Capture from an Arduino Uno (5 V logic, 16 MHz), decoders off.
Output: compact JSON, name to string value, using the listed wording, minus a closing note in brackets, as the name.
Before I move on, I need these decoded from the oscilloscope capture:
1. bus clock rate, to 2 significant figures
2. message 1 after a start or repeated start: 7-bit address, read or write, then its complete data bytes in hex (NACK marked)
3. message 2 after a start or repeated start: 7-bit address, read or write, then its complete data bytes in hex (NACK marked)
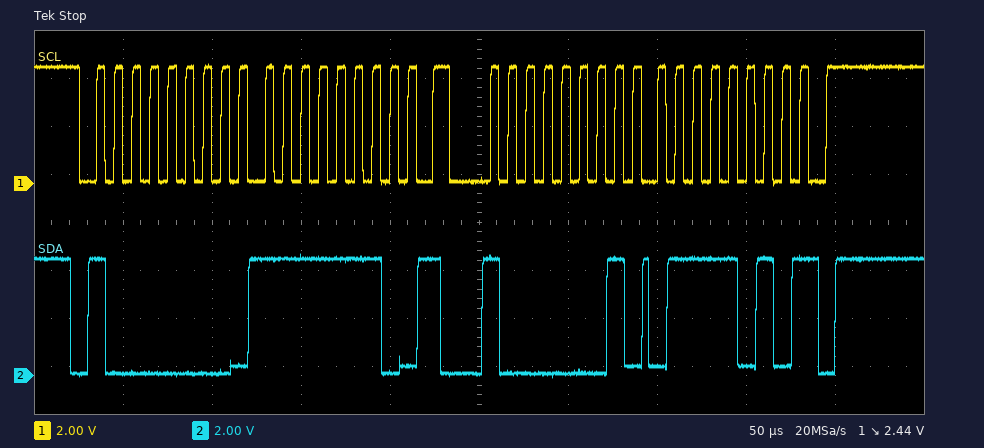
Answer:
{"bus clock rate, to 2 significant figures": "100 kHz", "message 1 after a start or repeated start: 7-bit address, read or write, then its complete data bytes in hex": "0x40 write: FE", "message 2 after a start or repeated start: 7-bit address, read or write, then its complete data bytes in hex": "0x40 read: 7A NACK"}
